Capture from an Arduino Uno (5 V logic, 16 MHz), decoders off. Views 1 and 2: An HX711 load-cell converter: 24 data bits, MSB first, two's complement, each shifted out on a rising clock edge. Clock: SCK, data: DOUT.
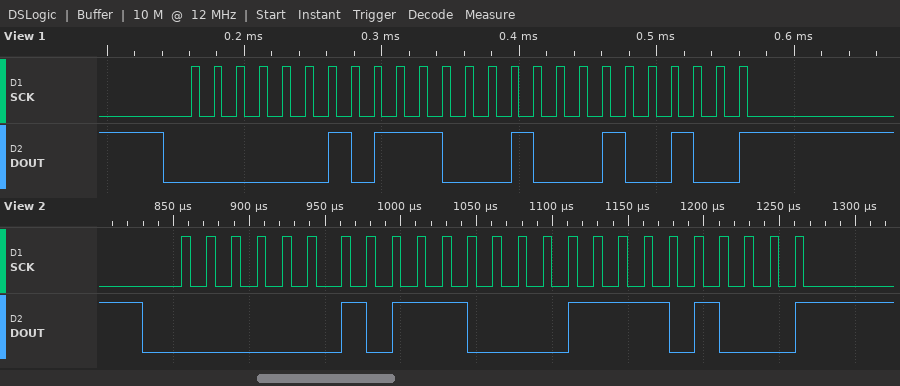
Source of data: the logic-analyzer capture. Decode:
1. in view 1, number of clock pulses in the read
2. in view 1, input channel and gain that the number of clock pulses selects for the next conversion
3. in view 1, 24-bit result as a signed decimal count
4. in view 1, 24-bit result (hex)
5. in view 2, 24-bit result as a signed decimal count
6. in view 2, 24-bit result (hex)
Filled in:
25
channel A, gain 128
188964
0x02E224
188904
0x02E1E8
